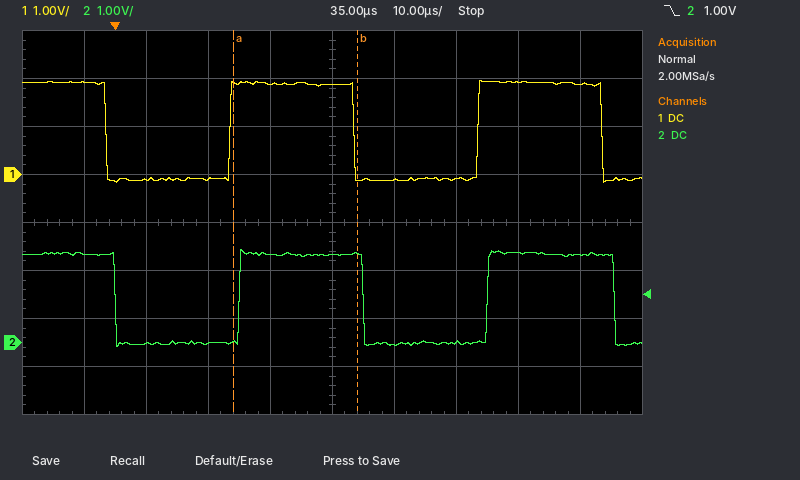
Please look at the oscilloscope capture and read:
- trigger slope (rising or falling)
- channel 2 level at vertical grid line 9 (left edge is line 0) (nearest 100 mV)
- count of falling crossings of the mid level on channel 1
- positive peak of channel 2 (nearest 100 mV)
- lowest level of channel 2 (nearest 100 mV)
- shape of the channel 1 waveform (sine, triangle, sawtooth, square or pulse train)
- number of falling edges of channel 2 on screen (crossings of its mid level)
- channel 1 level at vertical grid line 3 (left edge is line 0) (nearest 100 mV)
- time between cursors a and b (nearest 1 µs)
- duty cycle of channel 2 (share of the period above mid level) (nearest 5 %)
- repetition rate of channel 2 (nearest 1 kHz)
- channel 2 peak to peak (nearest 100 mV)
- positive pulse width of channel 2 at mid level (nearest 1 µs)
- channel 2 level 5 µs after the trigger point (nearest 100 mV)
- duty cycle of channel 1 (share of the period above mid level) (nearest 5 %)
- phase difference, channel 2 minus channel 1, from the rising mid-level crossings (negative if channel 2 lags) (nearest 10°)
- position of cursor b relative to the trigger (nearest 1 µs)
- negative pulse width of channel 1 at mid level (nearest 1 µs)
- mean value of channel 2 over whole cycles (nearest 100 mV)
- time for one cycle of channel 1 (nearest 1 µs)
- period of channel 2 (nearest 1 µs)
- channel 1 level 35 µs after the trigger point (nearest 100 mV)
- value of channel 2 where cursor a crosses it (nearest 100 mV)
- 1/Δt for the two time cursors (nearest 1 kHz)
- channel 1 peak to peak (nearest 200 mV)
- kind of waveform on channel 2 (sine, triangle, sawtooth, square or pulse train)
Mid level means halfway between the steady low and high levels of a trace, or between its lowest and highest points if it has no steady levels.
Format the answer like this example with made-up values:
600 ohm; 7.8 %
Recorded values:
falling; 1.8 V; 3; 1.9 V; -100 mV; square; 3; -100 mV; 20 µs; 50 %; 25 kHz; 2.0 V; 20 µs; 0.0 V; 50 %; -10°; +39 µs; 20 µs; 900 mV; 40 µs; 40 µs; 1.9 V; 0.0 V; 50 kHz; 2.2 V; square
